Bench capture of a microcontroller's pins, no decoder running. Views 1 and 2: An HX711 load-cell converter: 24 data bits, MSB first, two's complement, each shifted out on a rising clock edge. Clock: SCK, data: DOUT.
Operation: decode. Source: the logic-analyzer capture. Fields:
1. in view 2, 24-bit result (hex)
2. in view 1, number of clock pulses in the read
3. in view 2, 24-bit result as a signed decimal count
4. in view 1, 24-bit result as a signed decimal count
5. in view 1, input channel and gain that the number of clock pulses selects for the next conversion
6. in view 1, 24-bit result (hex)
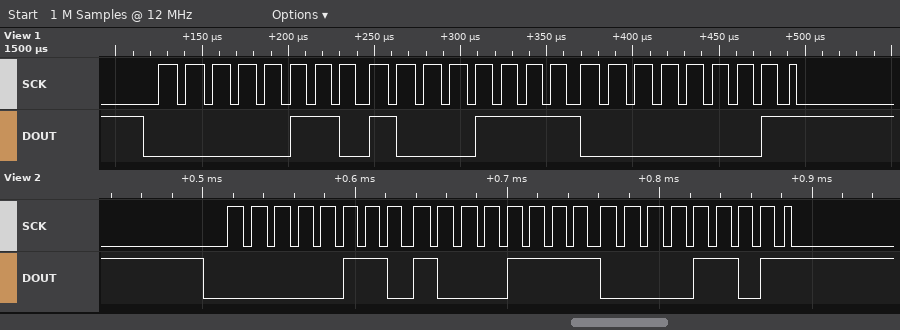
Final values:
0x068F0D
25
429837
429825
channel A, gain 128
0x068F01
